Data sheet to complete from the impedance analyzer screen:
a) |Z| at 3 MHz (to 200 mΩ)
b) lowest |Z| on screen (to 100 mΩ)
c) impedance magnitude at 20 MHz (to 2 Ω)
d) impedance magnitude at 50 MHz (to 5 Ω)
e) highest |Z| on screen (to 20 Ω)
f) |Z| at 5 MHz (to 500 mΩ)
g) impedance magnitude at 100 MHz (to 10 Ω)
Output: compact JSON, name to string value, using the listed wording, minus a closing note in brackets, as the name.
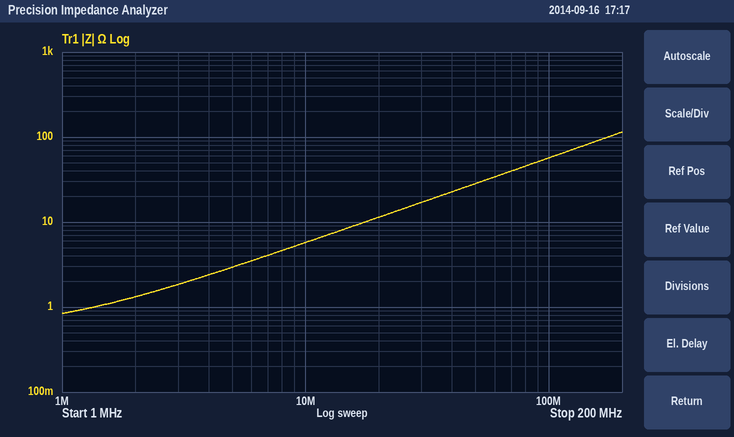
{"|Z| at 3 MHz": "1.8 Ω", "lowest |Z| on screen": "800 mΩ", "impedance magnitude at 20 MHz": "12 Ω", "impedance magnitude at 50 MHz": "30 Ω", "highest |Z| on screen": "120 Ω", "|Z| at 5 MHz": "3.0 Ω", "impedance magnitude at 100 MHz": "60 Ω"}
